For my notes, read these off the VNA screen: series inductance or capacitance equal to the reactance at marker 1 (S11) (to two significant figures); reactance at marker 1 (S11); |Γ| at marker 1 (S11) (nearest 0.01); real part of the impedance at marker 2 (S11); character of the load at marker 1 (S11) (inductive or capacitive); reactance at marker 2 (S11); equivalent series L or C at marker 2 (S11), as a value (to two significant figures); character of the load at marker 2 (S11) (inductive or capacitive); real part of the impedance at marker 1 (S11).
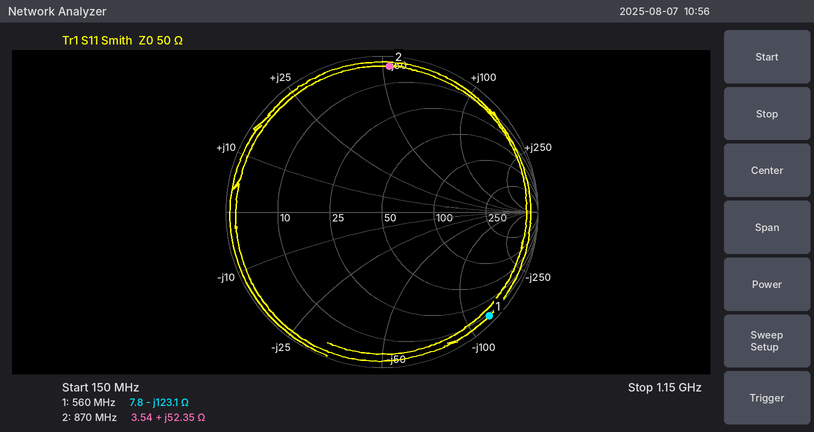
2.3 pF
-123.1 Ω
0.96
3.54 Ω
capacitive
+52.35 Ω
9.6 nH
inductive
7.8 Ω
